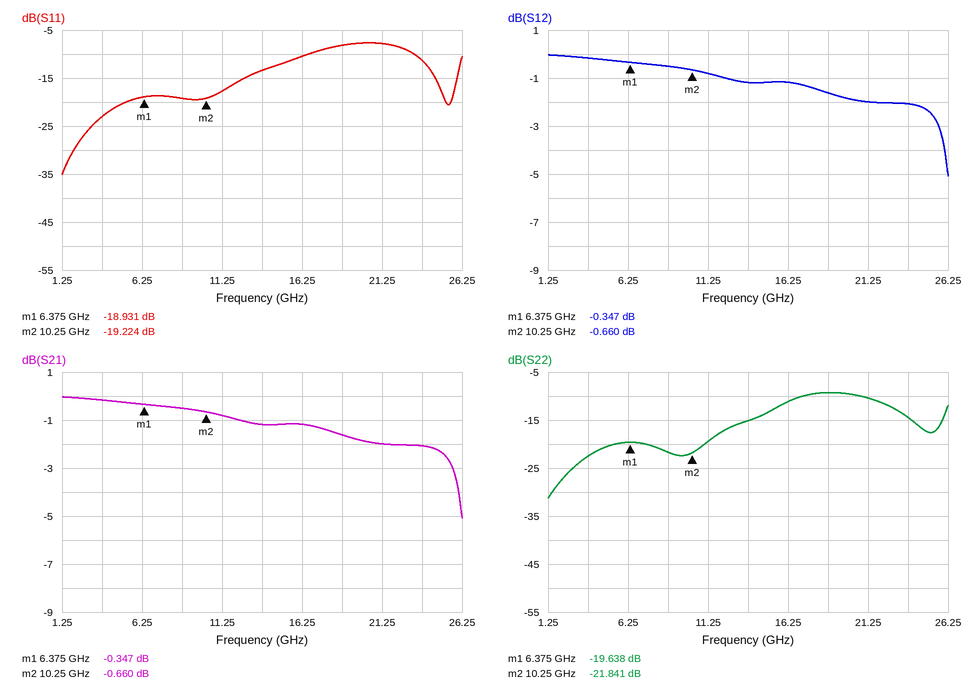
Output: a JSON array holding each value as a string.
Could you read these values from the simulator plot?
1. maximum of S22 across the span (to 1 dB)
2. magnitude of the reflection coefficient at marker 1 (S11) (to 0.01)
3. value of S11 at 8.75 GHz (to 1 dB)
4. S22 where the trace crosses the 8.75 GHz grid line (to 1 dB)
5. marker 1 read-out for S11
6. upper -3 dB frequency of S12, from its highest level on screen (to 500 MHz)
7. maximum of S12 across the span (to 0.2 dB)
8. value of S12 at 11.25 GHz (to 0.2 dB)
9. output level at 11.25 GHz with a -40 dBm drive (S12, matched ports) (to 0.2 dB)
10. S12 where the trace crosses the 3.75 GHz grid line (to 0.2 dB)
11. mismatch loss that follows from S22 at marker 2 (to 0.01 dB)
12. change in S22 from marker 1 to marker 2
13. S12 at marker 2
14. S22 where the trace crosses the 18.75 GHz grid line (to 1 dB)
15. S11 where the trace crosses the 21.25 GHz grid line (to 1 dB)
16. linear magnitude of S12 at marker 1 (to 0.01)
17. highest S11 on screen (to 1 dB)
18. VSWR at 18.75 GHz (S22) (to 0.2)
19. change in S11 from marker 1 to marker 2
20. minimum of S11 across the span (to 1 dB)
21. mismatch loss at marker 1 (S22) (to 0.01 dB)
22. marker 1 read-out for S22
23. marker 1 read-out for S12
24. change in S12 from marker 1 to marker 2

["-9 dB", "0.11", "-19 dB", "-22 dB", "-18.931 dB", "25.5 GHz", "0.0 dB", "-0.8 dB", "-40.8 dBm", "-0.2 dB", "0.03 dB", "-2.203 dB", "-0.660 dB", "-9 dB", "-8 dB", "0.96", "-8 dB", "2.0", "-0.293 dB", "-35 dB", "0.05 dB", "-19.638 dB", "-0.347 dB", "-0.313 dB"]
